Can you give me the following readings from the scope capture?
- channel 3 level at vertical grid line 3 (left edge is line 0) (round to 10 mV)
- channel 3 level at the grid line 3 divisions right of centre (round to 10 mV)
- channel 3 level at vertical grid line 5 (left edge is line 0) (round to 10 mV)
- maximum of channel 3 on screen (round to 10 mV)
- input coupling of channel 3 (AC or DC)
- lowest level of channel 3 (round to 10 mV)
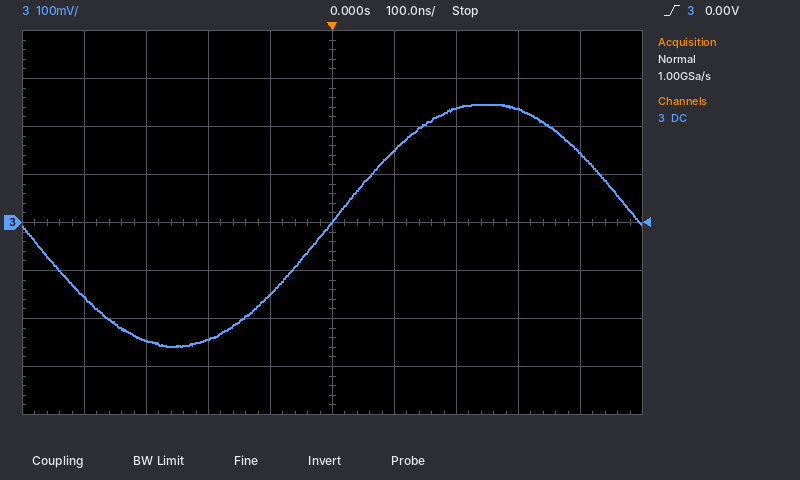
-240 mV
240 mV
0 mV
250 mV
DC
-260 mV
